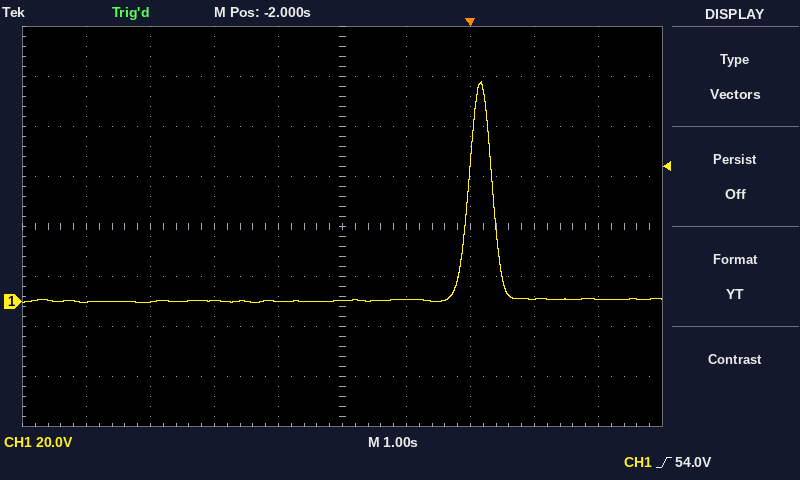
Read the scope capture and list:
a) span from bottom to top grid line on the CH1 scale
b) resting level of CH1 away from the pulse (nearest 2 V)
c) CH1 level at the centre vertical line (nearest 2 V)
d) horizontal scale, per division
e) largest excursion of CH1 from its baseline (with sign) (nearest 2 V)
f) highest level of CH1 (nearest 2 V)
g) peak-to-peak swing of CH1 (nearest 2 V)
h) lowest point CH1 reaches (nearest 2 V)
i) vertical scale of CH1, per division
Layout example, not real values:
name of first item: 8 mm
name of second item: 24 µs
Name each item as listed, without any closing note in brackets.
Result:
span from bottom to top grid line on the CH1 scale: 160 V
resting level of CH1 away from the pulse: 0 V
CH1 level at the centre vertical line: 0 V
horizontal scale, per division: 1 s
largest excursion of CH1 from its baseline (with sign): +88 V
highest level of CH1: 88 V
peak-to-peak swing of CH1: 88 V
lowest point CH1 reaches: 0 V
vertical scale of CH1, per division: 20 V
